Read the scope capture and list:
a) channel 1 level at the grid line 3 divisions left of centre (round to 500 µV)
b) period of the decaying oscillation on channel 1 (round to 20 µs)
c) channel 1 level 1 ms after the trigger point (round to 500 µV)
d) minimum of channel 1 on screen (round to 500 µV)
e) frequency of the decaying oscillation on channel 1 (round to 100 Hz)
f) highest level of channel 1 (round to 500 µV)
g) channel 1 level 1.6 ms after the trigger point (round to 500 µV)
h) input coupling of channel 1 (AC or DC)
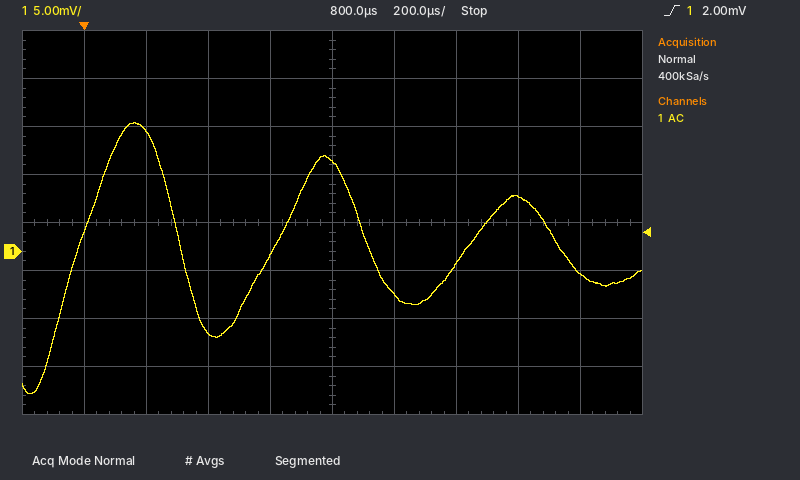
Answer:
12.5 mV
620 µs
-4.5 mV
-15.0 mV
1.6 kHz
13.5 mV
-2.5 mV
AC
